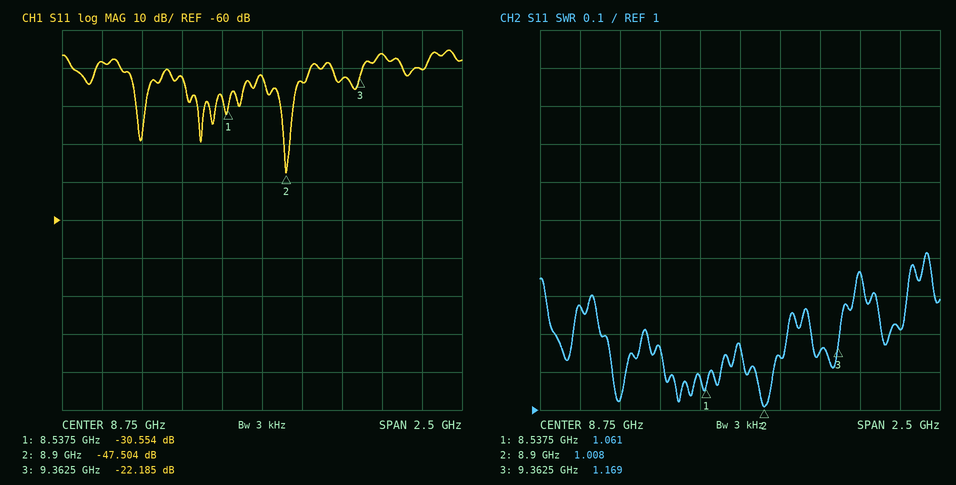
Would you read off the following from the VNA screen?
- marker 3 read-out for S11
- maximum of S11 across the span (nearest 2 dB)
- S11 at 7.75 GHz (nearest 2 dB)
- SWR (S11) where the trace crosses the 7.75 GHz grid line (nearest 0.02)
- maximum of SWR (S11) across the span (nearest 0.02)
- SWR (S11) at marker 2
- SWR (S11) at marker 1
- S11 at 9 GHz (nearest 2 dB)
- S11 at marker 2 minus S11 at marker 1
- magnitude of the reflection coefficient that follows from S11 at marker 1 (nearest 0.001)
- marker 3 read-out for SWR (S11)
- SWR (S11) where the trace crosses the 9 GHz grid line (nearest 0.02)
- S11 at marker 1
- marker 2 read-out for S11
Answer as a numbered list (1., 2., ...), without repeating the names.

1. -22.185 dB
2. -16 dB
3. -18 dB
4. 1.28
5. 1.42
6. 1.008
7. 1.061
8. -24 dB
9. -16.950 dB
10. 0.030
11. 1.169
12. 1.14
13. -30.554 dB
14. -47.504 dB
